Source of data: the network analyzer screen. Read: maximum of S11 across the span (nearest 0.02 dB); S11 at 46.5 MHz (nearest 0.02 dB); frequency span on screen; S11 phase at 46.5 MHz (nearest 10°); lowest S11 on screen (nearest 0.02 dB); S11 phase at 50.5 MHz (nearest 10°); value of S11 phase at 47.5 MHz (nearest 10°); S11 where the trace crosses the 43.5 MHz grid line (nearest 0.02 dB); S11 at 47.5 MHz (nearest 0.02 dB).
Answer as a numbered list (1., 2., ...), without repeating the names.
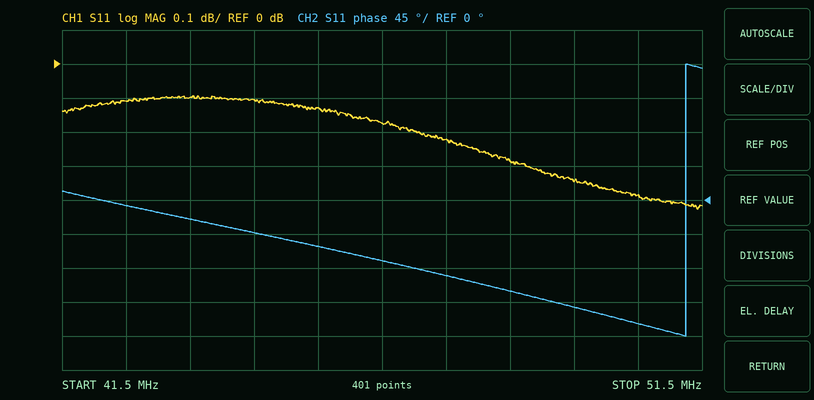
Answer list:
1. -0.10 dB
2. -0.18 dB
3. 10 MHz
4. -80°
5. -0.42 dB
6. -160°
7. -100°
8. -0.10 dB
9. -0.22 dB
